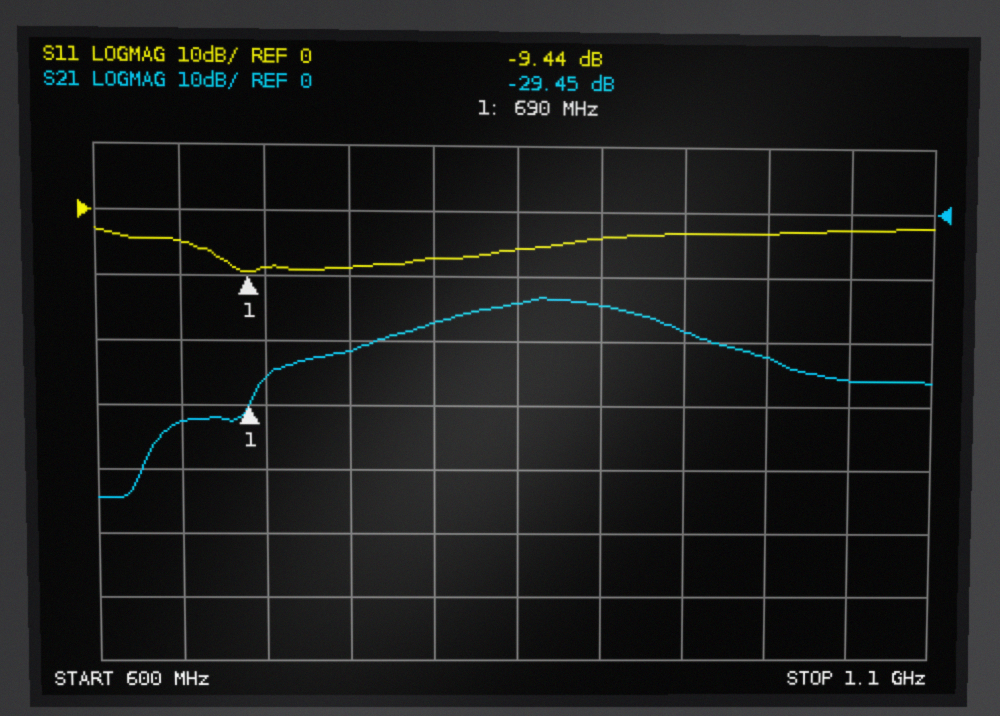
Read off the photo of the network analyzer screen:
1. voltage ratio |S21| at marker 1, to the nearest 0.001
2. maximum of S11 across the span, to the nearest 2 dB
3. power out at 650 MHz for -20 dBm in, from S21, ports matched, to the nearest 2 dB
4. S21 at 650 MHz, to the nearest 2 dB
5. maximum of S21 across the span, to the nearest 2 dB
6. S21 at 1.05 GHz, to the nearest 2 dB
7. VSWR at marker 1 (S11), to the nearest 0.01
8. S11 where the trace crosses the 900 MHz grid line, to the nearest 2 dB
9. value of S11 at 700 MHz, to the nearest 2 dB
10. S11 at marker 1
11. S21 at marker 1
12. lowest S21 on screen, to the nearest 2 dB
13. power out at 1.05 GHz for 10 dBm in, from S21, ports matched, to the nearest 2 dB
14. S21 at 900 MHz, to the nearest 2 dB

0.034
-2 dB
-52 dBm
-32 dB
-14 dB
-26 dB
2.02
-4 dB
-8 dB
-9.44 dB
-29.45 dB
-44 dB
-16 dBm
-14 dB
